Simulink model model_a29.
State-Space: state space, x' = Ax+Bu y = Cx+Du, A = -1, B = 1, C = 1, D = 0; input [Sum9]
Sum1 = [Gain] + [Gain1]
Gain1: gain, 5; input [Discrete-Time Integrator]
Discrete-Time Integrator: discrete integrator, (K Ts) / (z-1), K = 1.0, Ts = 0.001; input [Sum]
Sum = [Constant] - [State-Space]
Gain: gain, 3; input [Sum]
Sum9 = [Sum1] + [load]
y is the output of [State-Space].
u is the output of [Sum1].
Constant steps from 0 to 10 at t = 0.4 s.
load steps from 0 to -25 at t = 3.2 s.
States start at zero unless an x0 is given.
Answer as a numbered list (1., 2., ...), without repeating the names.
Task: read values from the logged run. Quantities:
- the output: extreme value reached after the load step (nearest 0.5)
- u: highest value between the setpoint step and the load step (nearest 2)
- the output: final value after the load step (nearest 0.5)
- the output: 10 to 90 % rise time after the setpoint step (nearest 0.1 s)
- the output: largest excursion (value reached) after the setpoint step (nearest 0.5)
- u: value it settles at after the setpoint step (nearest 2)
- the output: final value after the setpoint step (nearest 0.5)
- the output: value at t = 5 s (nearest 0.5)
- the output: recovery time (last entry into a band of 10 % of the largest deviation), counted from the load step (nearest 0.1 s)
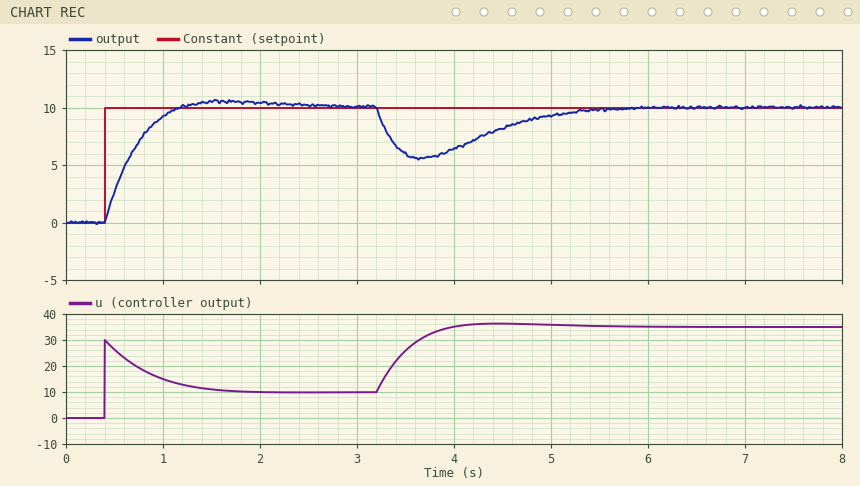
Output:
1. 5.5
2. 30
3. 10.0
4. 0.5 s
5. 10.5
6. 10
7. 10.0
8. 9.5
9. 2.0 s
